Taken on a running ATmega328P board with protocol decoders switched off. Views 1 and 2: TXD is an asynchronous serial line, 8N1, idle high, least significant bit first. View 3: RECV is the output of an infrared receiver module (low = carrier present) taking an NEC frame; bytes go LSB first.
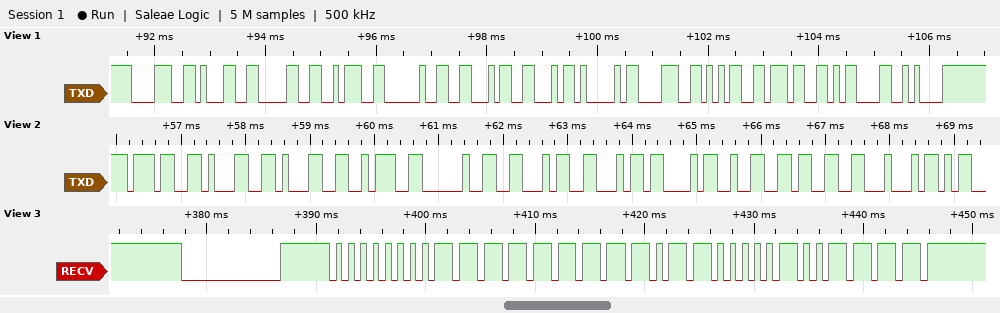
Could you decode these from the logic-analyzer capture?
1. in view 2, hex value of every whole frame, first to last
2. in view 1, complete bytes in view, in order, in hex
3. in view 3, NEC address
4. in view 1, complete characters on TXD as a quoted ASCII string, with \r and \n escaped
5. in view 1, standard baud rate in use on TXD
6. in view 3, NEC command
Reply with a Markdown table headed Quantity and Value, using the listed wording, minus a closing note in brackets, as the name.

| Quantity | Value |
|---|---|
| in view 2, hex value of every whole frame, first to last | 37 31 31 3A 20 46 46 43 32 33 44 |
| in view 1, complete bytes in view, in order, in hex | 38 31 30 3A 20 46 46 41 38 35 37 0D 0A |
| in view 3, NEC address | 0x00 |
| in view 1, complete characters on TXD as a quoted ASCII string, with \r and \n escaped | "810: FFA857\r\n" |
| in view 1, standard baud rate in use on TXD | 9600 baud |
| in view 3, NEC command | 0x0D |
